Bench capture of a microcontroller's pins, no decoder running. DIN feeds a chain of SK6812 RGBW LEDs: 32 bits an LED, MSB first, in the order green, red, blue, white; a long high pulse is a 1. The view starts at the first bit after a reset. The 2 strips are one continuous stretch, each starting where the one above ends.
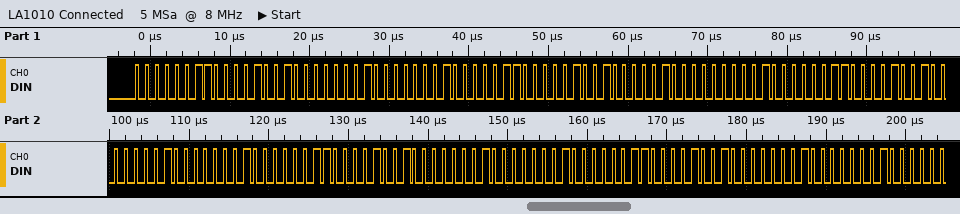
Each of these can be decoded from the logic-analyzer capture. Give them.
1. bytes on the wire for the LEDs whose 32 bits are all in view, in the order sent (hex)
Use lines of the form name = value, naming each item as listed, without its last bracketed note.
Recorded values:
bytes on the wire for the LEDs whose 32 bits are all in view, in the order sent = 03 09 01 01 06 09 04 01 03 09 01 01 03 09 01 01 03 09 01 01
